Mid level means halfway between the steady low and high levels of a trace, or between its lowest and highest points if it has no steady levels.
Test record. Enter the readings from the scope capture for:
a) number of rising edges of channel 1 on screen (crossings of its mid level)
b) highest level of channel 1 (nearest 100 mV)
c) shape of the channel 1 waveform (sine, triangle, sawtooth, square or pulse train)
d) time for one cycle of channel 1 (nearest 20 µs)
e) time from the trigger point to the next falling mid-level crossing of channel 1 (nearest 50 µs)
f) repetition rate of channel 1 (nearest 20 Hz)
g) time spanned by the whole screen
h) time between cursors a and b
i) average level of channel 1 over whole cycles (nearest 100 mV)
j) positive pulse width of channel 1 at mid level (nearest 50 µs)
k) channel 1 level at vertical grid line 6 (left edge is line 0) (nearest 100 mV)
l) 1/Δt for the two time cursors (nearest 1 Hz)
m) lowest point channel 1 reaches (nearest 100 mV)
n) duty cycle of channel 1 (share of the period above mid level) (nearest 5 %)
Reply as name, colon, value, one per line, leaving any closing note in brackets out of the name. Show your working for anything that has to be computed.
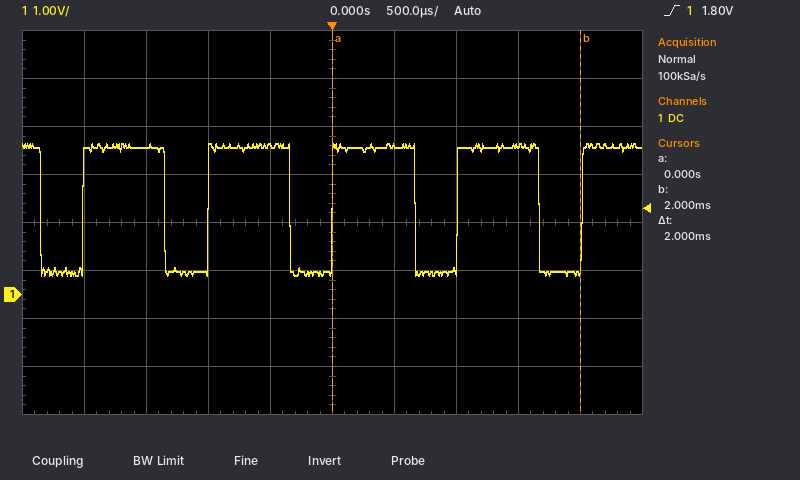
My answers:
number of rising edges of channel 1 on screen: 5
highest level of channel 1: 3.1 V
shape of the channel 1 waveform: pulse train
time for one cycle of channel 1: 1.00 ms
time from the trigger point to the next falling mid-level crossing of channel 1: 650 µs
repetition rate of channel 1: 1 / 1.00 ms ≈ 1.00 kHz
time spanned by the whole screen: 5 ms
time between cursors a and b: 2 ms
average level of channel 1 over whole cycles: 400 mV + 0.65 × (3.1 V − (400 mV)) ≈ 2.2 V
positive pulse width of channel 1 at mid level: 650 µs
channel 1 level at vertical grid line 6 (left edge is line 0): 3.1 V
1/Δt for the two time cursors: 1 / 2 ms ≈ 500 Hz
lowest point channel 1 reaches: 400 mV
duty cycle of channel 1 (share of the period above mid level): 650 µs / 1.00 ms ≈ 65 %
